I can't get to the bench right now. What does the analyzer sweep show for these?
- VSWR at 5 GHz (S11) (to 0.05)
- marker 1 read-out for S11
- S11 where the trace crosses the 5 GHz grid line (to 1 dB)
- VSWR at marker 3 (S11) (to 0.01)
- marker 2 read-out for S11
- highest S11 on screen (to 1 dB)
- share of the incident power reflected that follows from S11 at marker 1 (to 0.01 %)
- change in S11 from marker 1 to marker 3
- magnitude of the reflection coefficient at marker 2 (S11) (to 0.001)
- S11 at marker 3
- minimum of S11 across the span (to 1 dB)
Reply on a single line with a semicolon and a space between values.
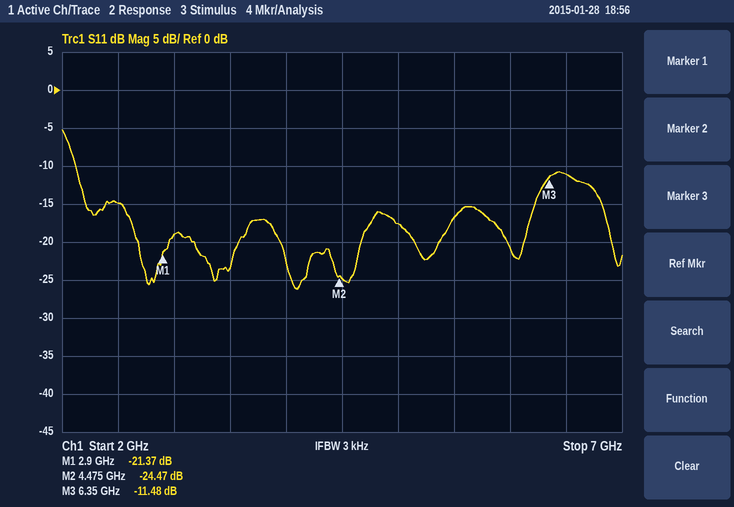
1.30; -21.37 dB; -18 dB; 1.73; -24.47 dB; -5 dB; 0.73 %; 9.89 dB; 0.060; -11.48 dB; -26 dB
